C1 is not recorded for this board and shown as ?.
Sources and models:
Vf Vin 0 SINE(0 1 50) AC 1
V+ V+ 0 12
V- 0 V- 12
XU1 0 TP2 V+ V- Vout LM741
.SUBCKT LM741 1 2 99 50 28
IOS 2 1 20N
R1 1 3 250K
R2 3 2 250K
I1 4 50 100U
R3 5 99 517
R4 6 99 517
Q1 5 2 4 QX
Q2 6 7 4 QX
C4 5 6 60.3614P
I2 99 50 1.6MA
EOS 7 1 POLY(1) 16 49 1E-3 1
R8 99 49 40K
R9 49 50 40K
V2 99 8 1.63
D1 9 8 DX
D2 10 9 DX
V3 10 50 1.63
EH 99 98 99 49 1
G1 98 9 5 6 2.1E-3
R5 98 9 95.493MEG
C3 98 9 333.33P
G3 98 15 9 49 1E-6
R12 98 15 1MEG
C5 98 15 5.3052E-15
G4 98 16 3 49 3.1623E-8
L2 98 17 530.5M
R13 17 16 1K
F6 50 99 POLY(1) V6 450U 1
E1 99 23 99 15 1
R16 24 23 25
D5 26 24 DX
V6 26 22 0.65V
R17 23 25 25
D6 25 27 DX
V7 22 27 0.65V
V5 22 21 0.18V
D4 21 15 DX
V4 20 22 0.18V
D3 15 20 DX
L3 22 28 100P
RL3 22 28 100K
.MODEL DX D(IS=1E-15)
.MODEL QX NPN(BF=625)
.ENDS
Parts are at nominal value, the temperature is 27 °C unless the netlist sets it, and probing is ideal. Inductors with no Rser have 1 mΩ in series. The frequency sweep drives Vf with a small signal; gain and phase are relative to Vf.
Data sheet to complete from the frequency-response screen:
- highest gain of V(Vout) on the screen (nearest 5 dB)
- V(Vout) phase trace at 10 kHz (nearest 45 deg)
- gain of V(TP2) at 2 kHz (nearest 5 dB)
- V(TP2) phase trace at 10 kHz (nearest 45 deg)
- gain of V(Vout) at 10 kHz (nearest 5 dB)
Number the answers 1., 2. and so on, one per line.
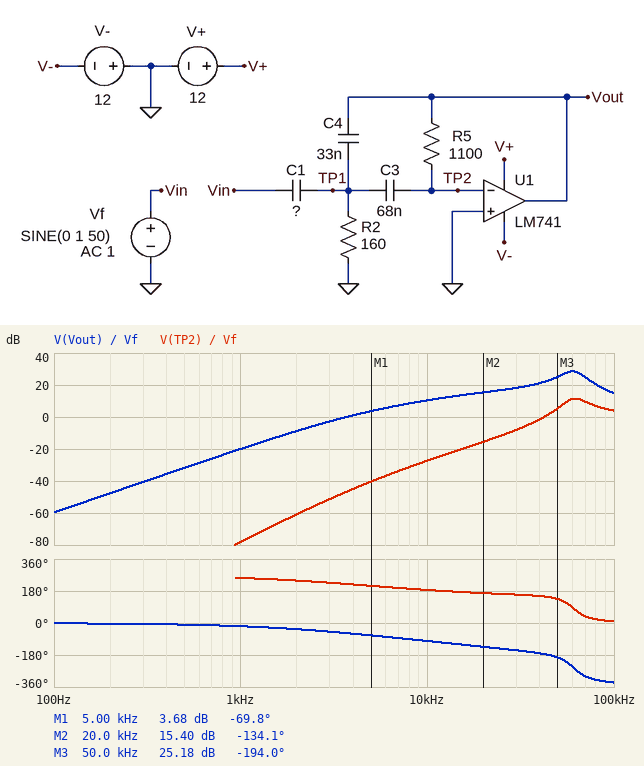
1. 30 dB
2. -90 deg
3. -60 dB
4. 180 deg
5. 10 dB
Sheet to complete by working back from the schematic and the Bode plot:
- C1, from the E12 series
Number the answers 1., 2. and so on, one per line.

1. 220 nF
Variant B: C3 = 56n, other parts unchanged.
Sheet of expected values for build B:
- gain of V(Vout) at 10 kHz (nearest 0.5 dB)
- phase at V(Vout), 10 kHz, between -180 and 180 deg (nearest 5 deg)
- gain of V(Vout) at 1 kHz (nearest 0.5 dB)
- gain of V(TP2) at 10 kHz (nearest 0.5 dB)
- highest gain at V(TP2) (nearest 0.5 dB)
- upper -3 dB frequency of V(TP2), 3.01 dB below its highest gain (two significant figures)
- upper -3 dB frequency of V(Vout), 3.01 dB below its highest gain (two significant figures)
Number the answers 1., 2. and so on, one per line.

1. 9.0 dB
2. -95 deg
3. -21.5 dB
4. -28.5 dB
5. 13.0 dB
6. 71 kHz
7. 68 kHz
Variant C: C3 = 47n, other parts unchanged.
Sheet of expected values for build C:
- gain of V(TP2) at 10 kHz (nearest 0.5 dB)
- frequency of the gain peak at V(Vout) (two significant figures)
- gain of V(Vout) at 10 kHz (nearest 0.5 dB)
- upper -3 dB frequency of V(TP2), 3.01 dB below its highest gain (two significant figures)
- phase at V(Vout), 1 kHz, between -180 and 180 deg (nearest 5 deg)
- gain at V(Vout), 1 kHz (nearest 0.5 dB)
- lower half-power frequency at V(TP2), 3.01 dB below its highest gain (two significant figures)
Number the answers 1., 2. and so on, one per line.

1. -29.5 dB
2. 61 kHz
3. 8.0 dB
4. 68 kHz
5. -15 deg
6. -23.0 dB
7. 57 kHz
